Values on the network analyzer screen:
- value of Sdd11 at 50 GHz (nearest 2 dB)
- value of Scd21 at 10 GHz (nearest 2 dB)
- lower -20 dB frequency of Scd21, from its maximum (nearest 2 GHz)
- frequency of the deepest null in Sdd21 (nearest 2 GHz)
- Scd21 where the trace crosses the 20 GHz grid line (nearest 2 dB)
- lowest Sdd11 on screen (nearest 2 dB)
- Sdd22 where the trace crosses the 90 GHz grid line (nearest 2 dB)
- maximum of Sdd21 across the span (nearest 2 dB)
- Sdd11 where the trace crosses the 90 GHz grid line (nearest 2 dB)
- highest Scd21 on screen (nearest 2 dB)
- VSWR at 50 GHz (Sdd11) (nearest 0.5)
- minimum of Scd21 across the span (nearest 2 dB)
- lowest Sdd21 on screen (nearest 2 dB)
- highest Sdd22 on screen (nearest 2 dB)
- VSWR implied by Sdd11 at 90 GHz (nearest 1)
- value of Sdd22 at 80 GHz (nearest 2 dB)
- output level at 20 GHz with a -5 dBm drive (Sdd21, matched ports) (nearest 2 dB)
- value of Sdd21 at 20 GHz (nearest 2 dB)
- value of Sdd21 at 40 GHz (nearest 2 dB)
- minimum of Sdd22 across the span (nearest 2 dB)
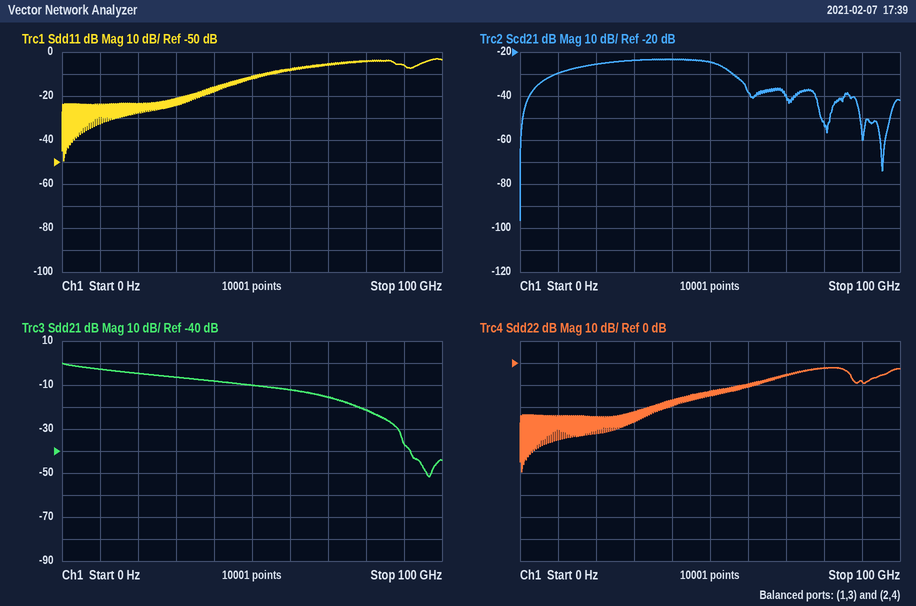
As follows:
-12 dB
-30 dB
2 GHz
96 GHz
-26 dB
-50 dB
-8 dB
0 dB
-6 dB
-24 dB
1.5
-96 dB
-52 dB
-2 dB
3
-2 dB
-10 dBm
-4 dB
-8 dB
-50 dB
